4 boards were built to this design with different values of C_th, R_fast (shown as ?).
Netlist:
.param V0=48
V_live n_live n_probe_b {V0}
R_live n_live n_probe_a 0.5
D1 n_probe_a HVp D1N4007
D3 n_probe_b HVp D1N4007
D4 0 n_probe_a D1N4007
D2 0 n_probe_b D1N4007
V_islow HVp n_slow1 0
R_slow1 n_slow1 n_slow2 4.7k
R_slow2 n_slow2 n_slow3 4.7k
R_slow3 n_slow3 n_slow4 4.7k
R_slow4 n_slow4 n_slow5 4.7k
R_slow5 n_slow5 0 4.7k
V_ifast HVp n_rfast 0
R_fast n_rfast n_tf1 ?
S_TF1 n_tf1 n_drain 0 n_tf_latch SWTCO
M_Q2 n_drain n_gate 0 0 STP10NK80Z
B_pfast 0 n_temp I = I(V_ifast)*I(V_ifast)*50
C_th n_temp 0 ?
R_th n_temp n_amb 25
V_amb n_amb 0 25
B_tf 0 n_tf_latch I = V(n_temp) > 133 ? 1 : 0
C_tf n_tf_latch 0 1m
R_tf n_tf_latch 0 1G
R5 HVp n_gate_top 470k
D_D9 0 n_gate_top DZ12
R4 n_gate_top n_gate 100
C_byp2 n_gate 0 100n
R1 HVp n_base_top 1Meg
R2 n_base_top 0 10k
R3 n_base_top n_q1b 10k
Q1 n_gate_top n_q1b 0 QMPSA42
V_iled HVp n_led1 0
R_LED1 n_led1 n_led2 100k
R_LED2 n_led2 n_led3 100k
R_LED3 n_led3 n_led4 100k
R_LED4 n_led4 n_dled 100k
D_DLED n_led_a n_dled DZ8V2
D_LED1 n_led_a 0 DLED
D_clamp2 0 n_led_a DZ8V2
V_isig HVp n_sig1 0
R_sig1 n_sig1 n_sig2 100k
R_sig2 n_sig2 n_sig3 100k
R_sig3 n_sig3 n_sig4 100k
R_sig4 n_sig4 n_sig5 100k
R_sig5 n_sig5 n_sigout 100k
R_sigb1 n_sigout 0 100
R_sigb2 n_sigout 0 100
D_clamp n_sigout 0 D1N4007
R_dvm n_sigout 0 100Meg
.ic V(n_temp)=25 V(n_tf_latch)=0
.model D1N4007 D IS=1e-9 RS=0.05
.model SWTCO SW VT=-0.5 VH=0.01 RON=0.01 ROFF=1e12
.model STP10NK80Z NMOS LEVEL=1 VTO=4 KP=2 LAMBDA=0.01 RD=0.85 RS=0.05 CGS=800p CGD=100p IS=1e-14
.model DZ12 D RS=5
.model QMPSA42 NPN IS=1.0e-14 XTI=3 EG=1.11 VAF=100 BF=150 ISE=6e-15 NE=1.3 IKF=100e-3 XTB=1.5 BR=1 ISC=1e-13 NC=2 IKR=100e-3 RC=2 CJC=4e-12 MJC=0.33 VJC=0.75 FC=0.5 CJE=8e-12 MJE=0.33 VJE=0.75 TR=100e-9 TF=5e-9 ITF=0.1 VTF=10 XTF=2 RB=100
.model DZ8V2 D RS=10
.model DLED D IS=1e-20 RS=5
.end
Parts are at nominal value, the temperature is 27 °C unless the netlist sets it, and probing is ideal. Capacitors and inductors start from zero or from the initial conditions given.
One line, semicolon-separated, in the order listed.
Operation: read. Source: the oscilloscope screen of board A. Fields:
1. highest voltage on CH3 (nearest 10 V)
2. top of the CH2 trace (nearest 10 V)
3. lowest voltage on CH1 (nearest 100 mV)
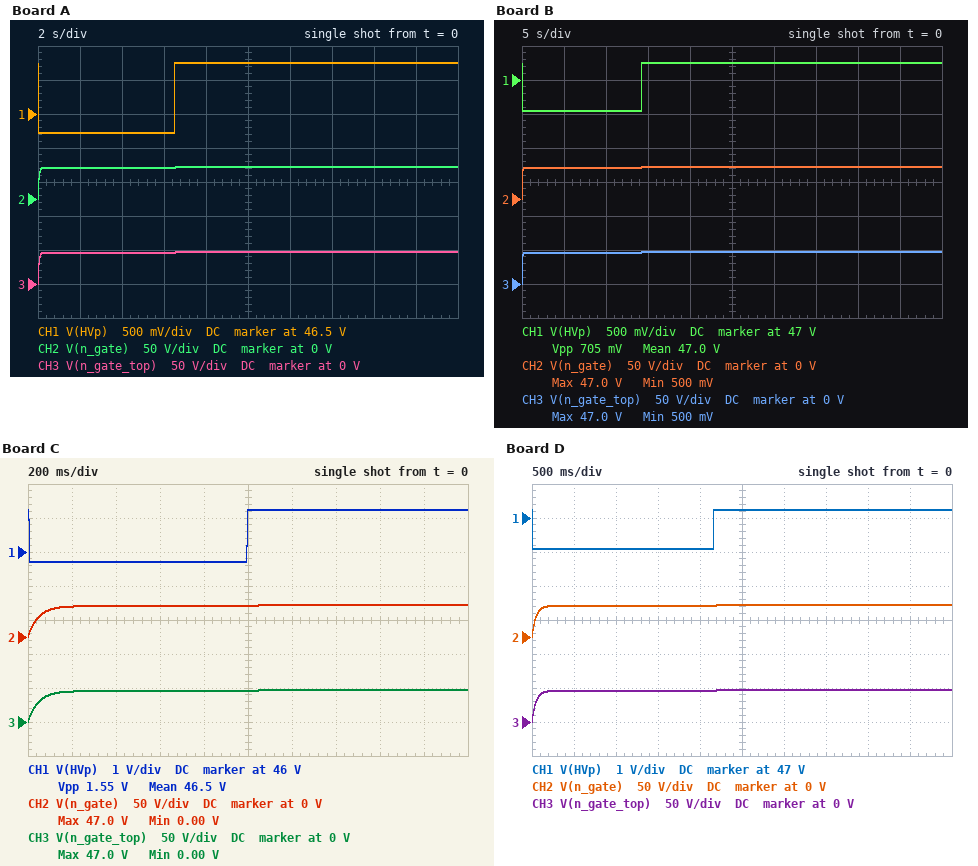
50 V; 50 V; 46.2 V
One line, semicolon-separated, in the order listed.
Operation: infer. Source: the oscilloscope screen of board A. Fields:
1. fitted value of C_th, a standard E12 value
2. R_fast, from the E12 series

3.9 F; 39 Ω
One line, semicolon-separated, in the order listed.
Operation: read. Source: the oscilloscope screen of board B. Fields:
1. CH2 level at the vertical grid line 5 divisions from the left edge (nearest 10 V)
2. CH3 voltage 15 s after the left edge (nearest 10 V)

50 V; 50 V
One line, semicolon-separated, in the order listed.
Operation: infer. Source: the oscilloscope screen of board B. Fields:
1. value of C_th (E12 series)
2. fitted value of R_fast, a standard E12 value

2.7 F; 68 Ω
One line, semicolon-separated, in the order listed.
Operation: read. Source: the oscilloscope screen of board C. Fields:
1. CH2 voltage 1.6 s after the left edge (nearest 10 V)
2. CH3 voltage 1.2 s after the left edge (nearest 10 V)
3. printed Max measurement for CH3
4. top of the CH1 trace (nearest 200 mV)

50 V; 50 V; 47.0 V; 47.2 V
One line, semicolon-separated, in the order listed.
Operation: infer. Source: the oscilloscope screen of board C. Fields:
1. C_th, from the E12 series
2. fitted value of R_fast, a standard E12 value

1.8 F; 22 Ω
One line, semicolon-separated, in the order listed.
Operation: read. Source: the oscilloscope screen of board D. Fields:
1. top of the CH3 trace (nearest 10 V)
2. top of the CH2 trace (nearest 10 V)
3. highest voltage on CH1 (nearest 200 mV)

50 V; 50 V; 47.2 V
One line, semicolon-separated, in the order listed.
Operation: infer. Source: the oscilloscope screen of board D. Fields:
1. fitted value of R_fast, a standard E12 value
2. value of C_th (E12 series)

33 Ω; 1.8 F
